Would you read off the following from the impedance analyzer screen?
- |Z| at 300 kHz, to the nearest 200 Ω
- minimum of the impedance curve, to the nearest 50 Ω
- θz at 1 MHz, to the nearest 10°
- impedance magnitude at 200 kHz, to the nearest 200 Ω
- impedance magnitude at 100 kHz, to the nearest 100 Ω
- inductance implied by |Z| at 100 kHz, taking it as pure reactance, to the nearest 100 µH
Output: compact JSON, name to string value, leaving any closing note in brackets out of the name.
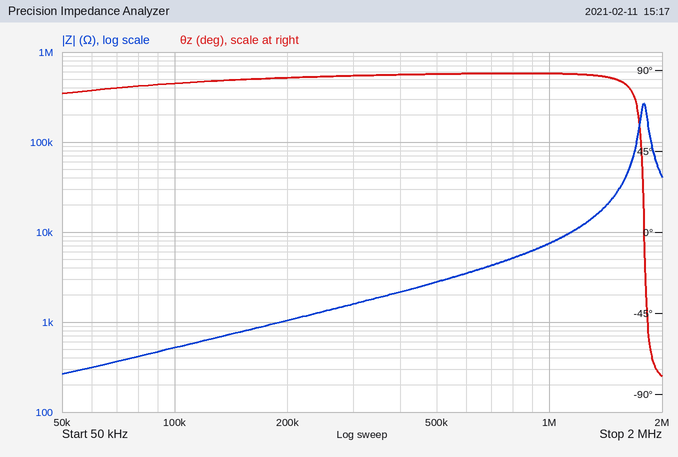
{"|Z| at 300 kHz, to the nearest 200 Ω": "1.6 kΩ", "minimum of the impedance curve, to the nearest 50 Ω": "250 Ω", "θz at 1 MHz, to the nearest 10°": "90°", "impedance magnitude at 200 kHz, to the nearest 200 Ω": "1.0 kΩ", "impedance magnitude at 100 kHz, to the nearest 100 Ω": "500 Ω", "inductance implied by |Z| at 100 kHz, taking it as pure reactance, to the nearest 100 µH": "800 µH"}
